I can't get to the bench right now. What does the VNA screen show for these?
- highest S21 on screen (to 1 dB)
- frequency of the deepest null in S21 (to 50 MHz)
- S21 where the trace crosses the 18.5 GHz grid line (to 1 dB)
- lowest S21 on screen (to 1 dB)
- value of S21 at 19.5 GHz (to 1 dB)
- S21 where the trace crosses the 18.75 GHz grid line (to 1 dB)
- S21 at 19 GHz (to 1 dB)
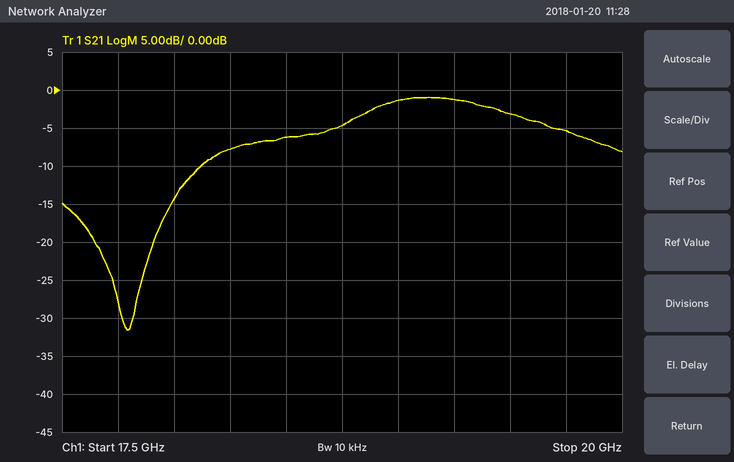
-1 dB
17.80 GHz
-6 dB
-32 dB
-3 dB
-5 dB
-1 dB
